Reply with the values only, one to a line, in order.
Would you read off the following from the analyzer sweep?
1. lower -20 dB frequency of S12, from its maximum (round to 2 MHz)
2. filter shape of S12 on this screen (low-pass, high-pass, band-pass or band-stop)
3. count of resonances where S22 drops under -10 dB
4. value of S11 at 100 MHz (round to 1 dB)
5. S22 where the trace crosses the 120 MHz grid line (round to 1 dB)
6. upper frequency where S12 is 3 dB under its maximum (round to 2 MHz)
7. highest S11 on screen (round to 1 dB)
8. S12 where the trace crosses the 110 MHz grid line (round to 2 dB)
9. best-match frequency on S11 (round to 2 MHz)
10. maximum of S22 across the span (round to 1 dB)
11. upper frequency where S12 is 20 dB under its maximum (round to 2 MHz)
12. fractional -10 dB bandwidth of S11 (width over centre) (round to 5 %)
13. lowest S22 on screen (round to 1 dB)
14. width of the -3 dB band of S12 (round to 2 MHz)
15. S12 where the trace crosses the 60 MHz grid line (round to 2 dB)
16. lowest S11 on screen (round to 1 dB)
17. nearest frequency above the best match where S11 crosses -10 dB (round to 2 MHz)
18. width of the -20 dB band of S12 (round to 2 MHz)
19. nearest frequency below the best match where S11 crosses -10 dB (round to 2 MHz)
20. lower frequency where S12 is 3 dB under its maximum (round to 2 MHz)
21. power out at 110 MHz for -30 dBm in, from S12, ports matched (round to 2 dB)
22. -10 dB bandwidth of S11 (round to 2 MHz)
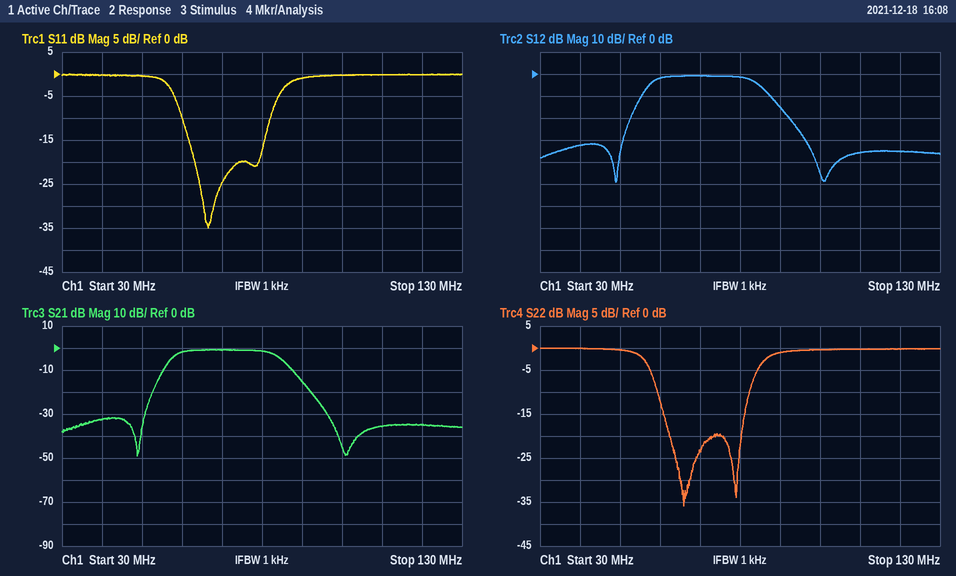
52 MHz
band-pass
2
0 dB
0 dB
84 MHz
0 dB
-36 dB
66 MHz
0 dB
92 MHz
30 %
-36 dB
26 MHz
-2 dB
-35 dB
82 MHz
40 MHz
60 MHz
58 MHz
-66 dBm
22 MHz
